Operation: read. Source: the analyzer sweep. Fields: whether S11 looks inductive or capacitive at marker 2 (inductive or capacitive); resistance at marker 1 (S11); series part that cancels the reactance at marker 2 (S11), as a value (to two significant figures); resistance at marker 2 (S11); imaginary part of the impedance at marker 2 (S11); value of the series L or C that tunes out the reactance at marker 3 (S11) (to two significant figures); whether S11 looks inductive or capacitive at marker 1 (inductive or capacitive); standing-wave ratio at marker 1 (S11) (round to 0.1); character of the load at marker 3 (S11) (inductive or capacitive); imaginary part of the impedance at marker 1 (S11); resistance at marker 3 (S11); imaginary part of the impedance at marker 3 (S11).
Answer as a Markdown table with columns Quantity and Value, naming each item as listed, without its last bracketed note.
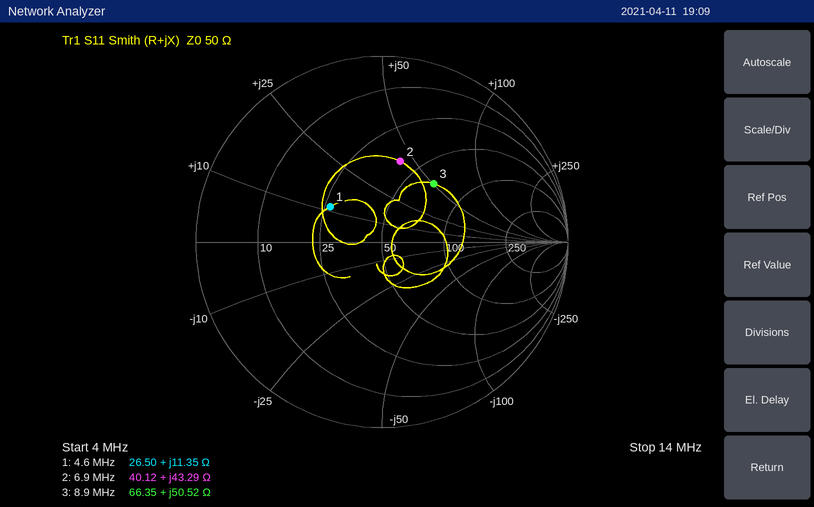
| Quantity | Value |
|---|---|
| whether S11 looks inductive or capacitive at marker 2 | inductive |
| resistance at marker 1 | 26.50 Ω |
| series part that cancels the reactance at marker 2 (S11), as a value | 530 pF |
| resistance at marker 2 | 40.12 Ω |
| imaginary part of the impedance at marker 2 | +43.29 Ω |
| value of the series L or C that tunes out the reactance at marker 3 (S11) | 350 pF |
| whether S11 looks inductive or capacitive at marker 1 | inductive |
| standing-wave ratio at marker 1 (S11) | 2.0 |
| character of the load at marker 3 (S11) | inductive |
| imaginary part of the impedance at marker 1 | +11.35 Ω |
| resistance at marker 3 | 66.35 Ω |
| imaginary part of the impedance at marker 3 | +50.52 Ω |
